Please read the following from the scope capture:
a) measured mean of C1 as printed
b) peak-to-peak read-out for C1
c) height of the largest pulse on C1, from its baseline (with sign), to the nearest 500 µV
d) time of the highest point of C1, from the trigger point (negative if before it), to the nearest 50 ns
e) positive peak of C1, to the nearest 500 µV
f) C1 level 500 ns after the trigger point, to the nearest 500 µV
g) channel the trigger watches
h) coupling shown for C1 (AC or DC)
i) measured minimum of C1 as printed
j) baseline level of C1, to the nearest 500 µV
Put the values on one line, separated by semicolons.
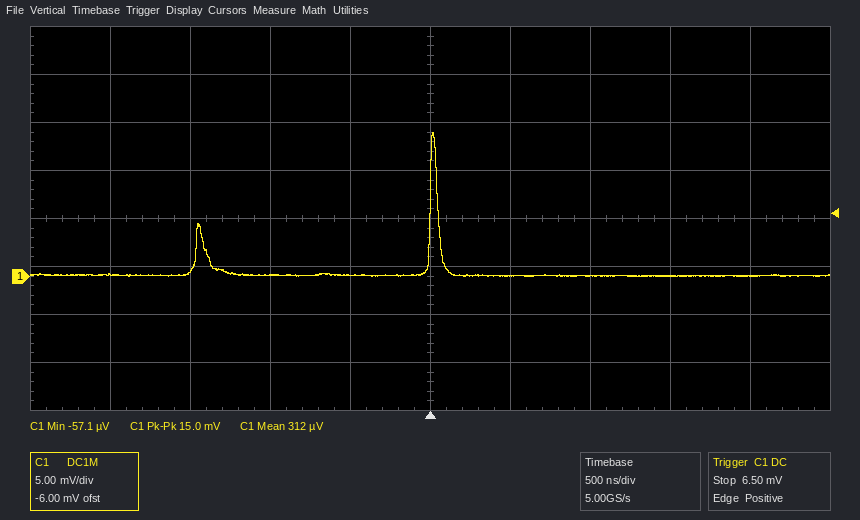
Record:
312 µV; 15.0 mV; +15.0 mV; 0 ns; 15.0 mV; 0.0 mV; C1; DC; -57.1 µV; 0.0 mV
